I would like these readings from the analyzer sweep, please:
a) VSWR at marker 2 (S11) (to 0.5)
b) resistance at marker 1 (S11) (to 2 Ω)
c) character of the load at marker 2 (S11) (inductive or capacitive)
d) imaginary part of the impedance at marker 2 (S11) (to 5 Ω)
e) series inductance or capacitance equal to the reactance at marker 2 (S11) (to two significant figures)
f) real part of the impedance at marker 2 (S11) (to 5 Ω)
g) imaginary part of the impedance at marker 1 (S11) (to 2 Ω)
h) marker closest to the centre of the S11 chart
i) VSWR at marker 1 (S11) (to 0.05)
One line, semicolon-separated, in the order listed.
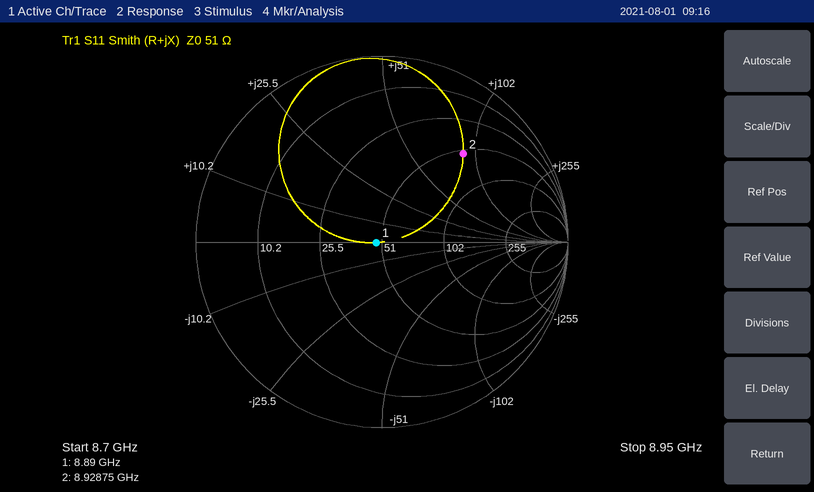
4.5; 48 Ω; inductive; +90 Ω; 1.6 nH; 55 Ω; 0 Ω; marker 1; 1.05
